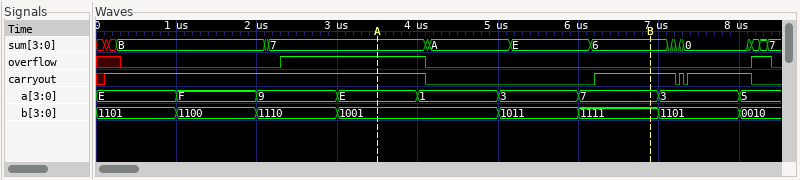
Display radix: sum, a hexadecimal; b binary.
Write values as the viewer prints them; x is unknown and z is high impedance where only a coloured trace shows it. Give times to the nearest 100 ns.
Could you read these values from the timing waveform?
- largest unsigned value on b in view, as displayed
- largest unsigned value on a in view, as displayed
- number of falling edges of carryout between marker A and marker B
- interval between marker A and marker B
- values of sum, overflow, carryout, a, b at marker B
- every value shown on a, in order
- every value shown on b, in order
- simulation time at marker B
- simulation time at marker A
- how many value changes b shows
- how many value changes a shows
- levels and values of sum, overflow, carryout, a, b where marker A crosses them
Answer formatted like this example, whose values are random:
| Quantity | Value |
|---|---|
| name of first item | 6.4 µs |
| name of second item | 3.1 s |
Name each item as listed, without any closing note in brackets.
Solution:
| Quantity | Value |
|---|---|
| largest unsigned value on b in view, as displayed | 1111 |
| largest unsigned value on a in view, as displayed | F |
| number of falling edges of carryout between marker A and marker B | 1 |
| interval between marker A and marker B | 3400 ns |
| values of sum, overflow, carryout, a, b at marker B | sum=6, overflow=0, carryout=1, a=7, b=1111 |
| every value shown on a, in order | E, F, 9, E, 1, 3, 7, 3, 5 |
| every value shown on b, in order | 1101, 1100, 1110, 1001, 1011, 1111, 1101, 0010 |
| simulation time at marker B | 6900 ns |
| simulation time at marker A | 3500 ns |
| how many value changes b shows | 7 |
| how many value changes a shows | 8 |
| levels and values of sum, overflow, carryout, a, b where marker A crosses them | sum=7, overflow=1, carryout=1, a=E, b=1001 |
